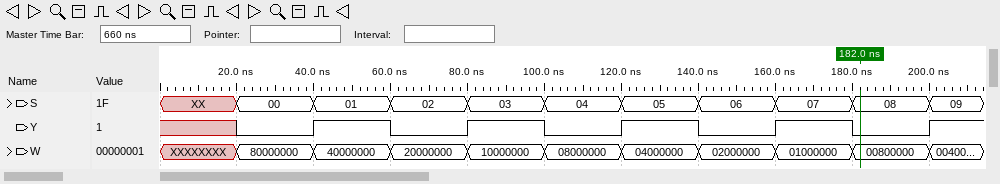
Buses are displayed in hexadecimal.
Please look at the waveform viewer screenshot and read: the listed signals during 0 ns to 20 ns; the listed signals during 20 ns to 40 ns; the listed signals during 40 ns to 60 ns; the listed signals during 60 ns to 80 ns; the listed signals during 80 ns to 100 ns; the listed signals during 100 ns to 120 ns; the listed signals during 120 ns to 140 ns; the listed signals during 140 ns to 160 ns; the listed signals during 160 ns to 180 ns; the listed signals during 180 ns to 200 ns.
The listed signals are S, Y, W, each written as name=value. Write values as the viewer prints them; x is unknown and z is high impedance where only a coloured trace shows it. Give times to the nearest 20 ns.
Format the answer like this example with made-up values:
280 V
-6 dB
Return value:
S=XX, Y=x, W=XXXXXXXX
S=00, Y=0, W=80000000
S=01, Y=1, W=40000000
S=02, Y=0, W=20000000
S=03, Y=1, W=10000000
S=04, Y=0, W=08000000
S=05, Y=1, W=04000000
S=06, Y=0, W=02000000
S=07, Y=1, W=01000000
S=08, Y=0, W=00800000
